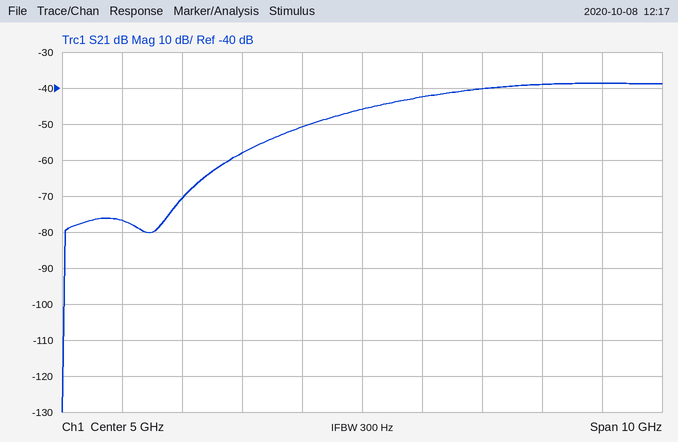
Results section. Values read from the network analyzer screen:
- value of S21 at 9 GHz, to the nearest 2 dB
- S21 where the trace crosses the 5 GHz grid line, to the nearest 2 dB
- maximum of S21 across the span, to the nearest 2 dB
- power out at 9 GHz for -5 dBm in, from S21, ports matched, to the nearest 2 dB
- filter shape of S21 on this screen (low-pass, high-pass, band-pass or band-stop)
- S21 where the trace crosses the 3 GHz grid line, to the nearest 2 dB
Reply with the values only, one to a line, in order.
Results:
-38 dB
-46 dB
-38 dB
-44 dBm
high-pass
-58 dB
